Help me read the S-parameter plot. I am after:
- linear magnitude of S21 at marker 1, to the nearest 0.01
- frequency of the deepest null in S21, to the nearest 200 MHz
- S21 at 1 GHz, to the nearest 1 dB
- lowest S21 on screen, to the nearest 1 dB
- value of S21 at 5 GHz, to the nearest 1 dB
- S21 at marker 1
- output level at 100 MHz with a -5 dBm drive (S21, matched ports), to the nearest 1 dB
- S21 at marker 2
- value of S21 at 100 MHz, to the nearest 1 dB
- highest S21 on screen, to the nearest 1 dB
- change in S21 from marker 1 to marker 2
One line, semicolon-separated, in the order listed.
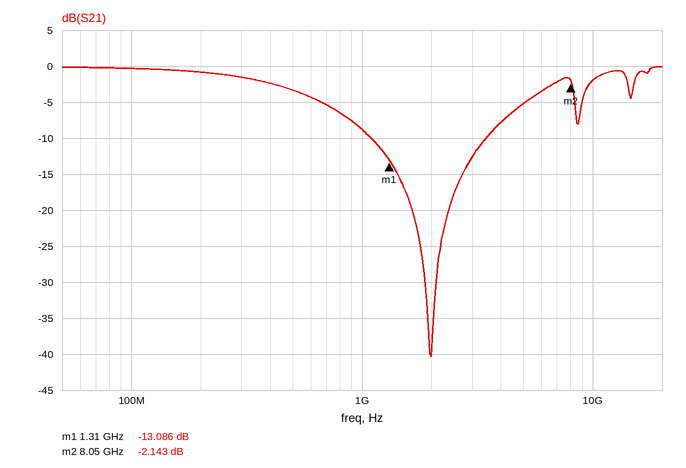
0.22; 2.0 GHz; -9 dB; -40 dB; -5 dB; -13.086 dB; -5 dBm; -2.143 dB; 0 dB; 0 dB; 10.943 dB
